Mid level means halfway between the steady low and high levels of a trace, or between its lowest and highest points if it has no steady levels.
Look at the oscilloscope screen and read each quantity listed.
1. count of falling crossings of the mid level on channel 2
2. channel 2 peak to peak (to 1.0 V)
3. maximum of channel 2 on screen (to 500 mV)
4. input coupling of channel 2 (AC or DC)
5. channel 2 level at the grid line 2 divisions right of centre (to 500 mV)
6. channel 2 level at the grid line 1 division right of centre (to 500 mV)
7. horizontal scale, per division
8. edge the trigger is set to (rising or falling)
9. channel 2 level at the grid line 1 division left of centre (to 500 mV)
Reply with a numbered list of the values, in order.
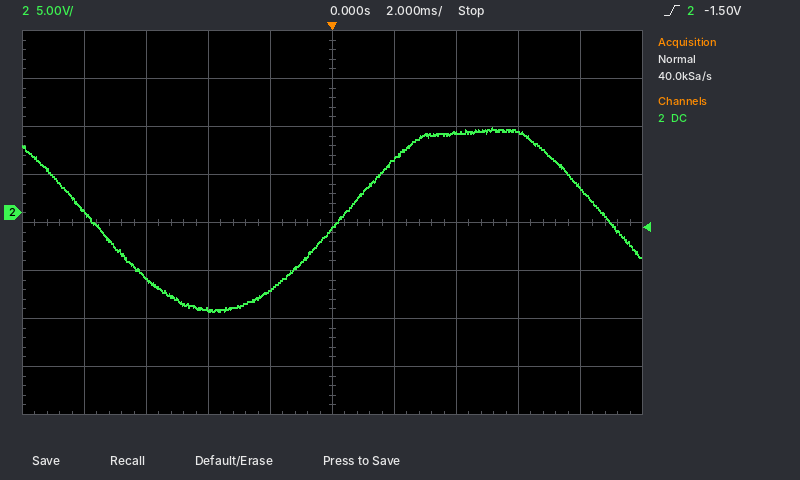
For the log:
1. 2
2. 19.0 V
3. 9.0 V
4. DC
5. 8.5 V
6. 5.5 V
7. 2 ms
8. rising
9. -8.0 V
